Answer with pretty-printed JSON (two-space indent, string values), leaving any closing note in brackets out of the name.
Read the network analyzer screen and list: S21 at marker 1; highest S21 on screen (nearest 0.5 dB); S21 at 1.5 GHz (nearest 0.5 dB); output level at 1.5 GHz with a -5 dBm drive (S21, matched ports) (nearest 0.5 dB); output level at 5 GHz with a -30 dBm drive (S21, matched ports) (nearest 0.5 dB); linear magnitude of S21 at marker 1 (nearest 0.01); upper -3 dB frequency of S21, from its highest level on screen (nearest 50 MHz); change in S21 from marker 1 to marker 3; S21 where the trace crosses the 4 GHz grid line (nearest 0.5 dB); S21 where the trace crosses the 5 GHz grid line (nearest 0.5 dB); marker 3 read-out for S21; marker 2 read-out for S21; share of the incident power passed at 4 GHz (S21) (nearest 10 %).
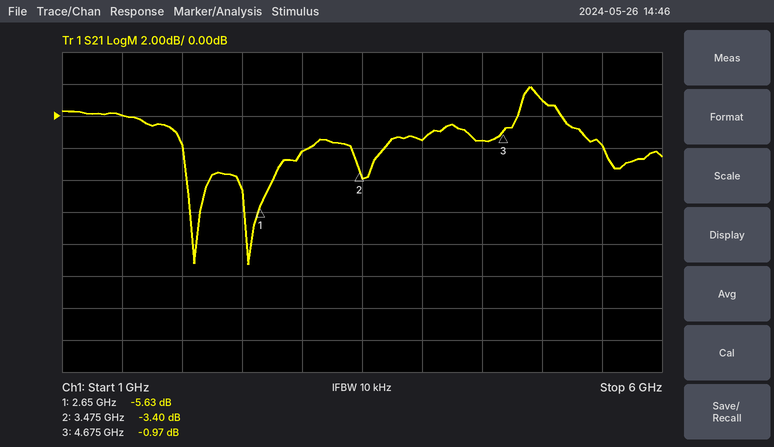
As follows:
{
  "S21 at marker 1": "-5.63 dB",
  "highest S21 on screen": "2.0 dB",
  "S21 at 1.5 GHz": "0.0 dB",
  "output level at 1.5 GHz with a -5 dBm drive (S21, matched ports)": "-5.0 dBm",
  "output level at 5 GHz with a -30 dBm drive (S21, matched ports)": "-29.0 dBm",
  "linear magnitude of S21 at marker 1": "0.52",
  "upper -3 dB frequency of S21, from its highest level on screen": "5.35 GHz",
  "change in S21 from marker 1 to marker 3": "4.66 dB",
  "S21 where the trace crosses the 4 GHz grid line": "-1.5 dB",
  "S21 where the trace crosses the 5 GHz grid line": "1.0 dB",
  "marker 3 read-out for S21": "-0.97 dB",
  "marker 2 read-out for S21": "-3.40 dB",
  "share of the incident power passed at 4 GHz (S21)": "70 %"
}
